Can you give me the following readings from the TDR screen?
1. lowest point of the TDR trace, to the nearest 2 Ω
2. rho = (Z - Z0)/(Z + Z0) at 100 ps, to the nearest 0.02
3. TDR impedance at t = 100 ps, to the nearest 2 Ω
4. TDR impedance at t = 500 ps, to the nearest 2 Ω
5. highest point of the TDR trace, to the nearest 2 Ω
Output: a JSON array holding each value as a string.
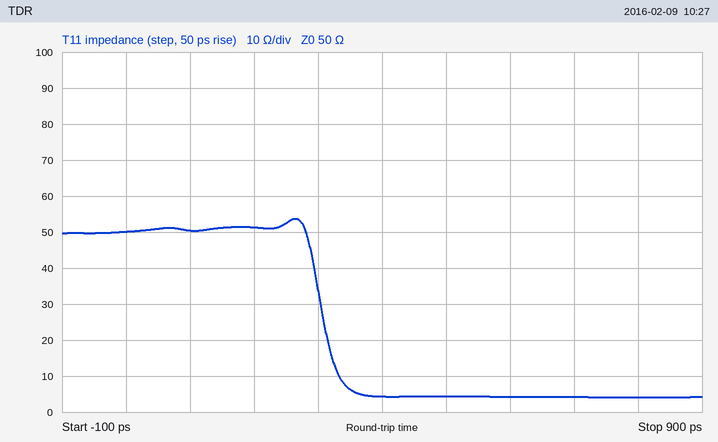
["4 Ω", "0.00", "50 Ω", "4 Ω", "54 Ω"]
